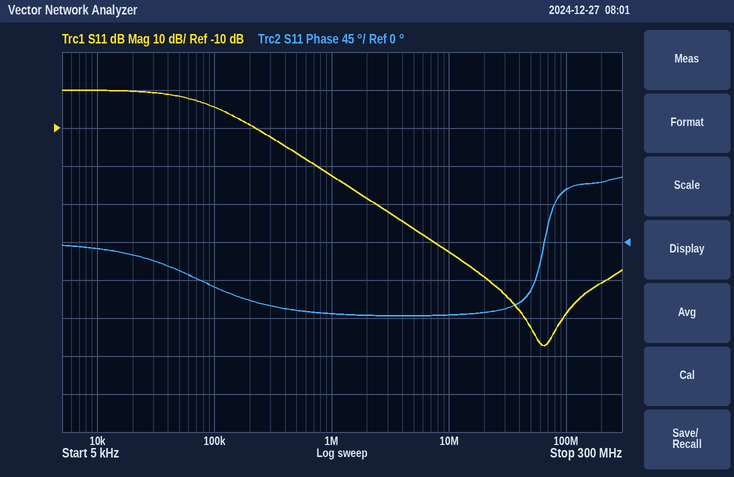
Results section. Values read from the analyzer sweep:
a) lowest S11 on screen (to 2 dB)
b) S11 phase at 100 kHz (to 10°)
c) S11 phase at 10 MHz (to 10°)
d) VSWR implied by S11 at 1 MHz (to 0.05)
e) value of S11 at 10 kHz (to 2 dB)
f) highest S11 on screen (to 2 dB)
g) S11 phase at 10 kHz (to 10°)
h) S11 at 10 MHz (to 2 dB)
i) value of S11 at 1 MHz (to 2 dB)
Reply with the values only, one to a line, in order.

-68 dB
-50°
-90°
1.15
0 dB
0 dB
-10°
-42 dB
-22 dB
